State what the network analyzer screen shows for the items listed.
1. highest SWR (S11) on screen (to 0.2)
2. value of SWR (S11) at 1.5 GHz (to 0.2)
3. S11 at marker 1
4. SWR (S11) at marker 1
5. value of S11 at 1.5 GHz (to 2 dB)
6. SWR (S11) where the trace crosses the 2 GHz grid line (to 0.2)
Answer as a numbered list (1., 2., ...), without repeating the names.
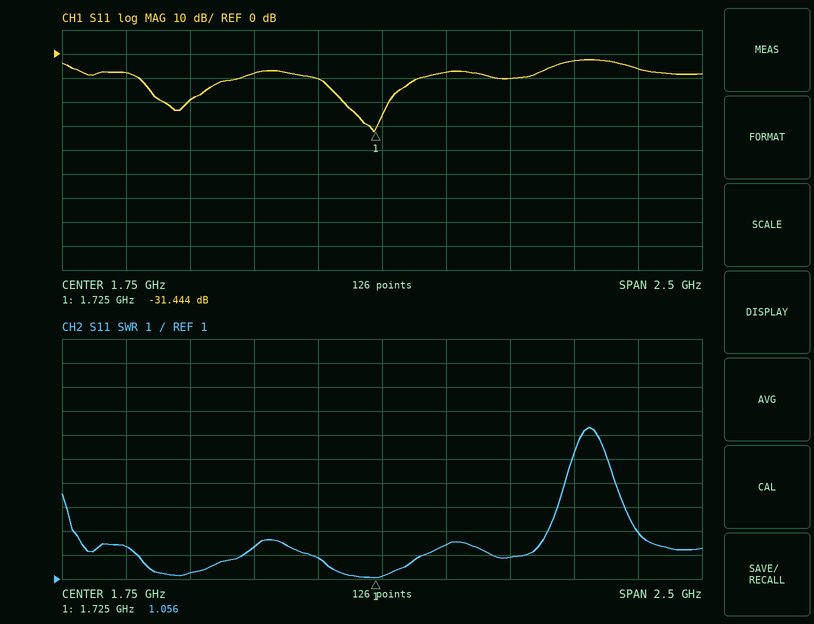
1. 7.4
2. 1.8
3. -31.444 dB
4. 1.056
5. -10 dB
6. 2.4
